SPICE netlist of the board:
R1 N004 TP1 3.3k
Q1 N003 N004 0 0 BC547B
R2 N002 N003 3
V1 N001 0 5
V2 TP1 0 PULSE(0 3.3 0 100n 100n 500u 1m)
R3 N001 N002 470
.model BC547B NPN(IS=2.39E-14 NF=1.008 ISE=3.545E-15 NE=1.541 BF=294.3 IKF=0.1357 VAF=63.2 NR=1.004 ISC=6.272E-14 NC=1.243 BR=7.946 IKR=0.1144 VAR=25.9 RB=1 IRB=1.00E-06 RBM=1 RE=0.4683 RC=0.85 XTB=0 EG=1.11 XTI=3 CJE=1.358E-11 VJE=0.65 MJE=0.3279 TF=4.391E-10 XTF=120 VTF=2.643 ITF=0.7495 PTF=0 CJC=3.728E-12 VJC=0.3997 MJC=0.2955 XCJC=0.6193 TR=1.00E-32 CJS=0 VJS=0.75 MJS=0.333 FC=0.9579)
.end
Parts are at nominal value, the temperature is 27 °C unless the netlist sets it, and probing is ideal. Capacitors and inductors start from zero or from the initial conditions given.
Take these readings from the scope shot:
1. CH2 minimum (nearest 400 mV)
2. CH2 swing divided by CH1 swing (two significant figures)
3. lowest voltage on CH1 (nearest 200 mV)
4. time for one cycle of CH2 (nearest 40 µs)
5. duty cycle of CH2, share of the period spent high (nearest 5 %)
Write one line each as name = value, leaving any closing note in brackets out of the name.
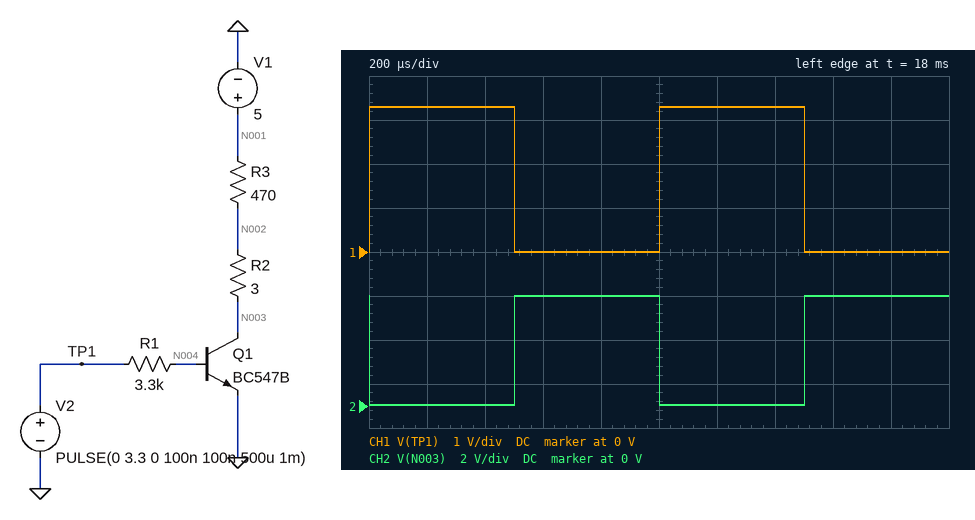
CH2 minimum = 0 V
CH2 swing divided by CH1 swing = 1.5
lowest voltage on CH1 = 0 V
time for one cycle of CH2 = 1.00 ms
duty cycle of CH2, share of the period spent high = 50 %
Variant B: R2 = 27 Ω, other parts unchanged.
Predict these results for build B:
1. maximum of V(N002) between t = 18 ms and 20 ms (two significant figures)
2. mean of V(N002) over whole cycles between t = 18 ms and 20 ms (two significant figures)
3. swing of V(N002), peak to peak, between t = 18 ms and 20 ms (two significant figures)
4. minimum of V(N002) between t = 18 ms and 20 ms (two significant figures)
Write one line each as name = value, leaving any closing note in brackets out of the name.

maximum of V(N002) between t = 18 ms and 20 ms = 5.0 V
mean of V(N002) over whole cycles between t = 18 ms and 20 ms = 2.7 V
swing of V(N002), peak to peak, between t = 18 ms and 20 ms = 4.7 V
minimum of V(N002) between t = 18 ms and 20 ms = 320 mV
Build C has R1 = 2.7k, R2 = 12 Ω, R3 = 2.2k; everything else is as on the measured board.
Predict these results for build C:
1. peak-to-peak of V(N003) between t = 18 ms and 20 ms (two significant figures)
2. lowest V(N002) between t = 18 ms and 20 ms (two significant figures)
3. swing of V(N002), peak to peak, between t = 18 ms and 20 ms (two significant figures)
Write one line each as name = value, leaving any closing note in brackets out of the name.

peak-to-peak of V(N003) between t = 18 ms and 20 ms = 5.0 V
lowest V(N002) between t = 18 ms and 20 ms = 45 mV
swing of V(N002), peak to peak, between t = 18 ms and 20 ms = 5.0 V
